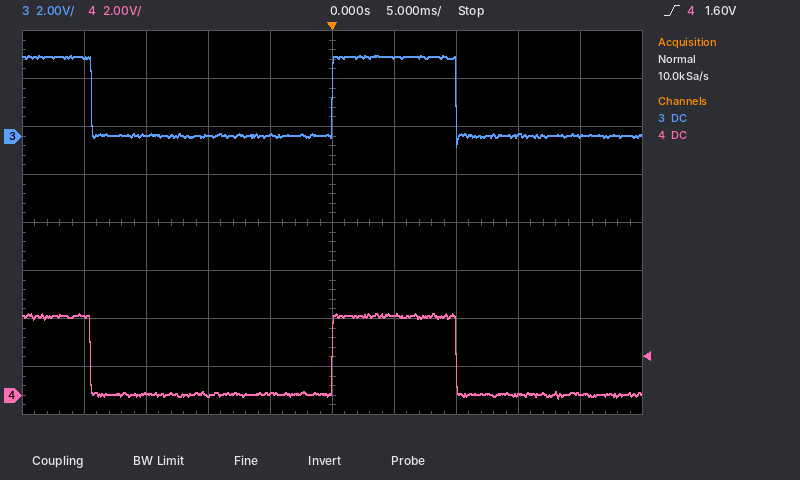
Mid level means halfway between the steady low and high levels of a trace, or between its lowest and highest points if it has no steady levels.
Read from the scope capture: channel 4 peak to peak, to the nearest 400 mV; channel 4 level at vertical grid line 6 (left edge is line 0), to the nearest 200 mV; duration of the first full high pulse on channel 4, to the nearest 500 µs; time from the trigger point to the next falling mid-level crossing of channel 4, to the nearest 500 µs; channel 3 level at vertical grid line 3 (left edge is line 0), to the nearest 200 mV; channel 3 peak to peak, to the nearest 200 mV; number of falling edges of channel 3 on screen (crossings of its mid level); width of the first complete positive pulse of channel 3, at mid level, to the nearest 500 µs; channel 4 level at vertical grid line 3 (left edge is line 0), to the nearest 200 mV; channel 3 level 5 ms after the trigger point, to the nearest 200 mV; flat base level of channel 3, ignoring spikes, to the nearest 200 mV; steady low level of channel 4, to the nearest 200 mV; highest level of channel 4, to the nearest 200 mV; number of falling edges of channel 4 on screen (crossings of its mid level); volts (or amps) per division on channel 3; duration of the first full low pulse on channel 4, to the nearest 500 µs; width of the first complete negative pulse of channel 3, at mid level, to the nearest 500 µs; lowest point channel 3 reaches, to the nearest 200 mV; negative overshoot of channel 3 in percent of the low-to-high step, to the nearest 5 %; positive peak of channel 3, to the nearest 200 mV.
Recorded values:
3.6 V
3.4 V
10.0 ms
10.0 ms
0.0 V
3.8 V
2
10.0 ms
0.0 V
3.2 V
0.0 V
0.0 V
3.4 V
2
2 V
19.5 ms
19.5 ms
-400 mV
15 %
3.4 V
